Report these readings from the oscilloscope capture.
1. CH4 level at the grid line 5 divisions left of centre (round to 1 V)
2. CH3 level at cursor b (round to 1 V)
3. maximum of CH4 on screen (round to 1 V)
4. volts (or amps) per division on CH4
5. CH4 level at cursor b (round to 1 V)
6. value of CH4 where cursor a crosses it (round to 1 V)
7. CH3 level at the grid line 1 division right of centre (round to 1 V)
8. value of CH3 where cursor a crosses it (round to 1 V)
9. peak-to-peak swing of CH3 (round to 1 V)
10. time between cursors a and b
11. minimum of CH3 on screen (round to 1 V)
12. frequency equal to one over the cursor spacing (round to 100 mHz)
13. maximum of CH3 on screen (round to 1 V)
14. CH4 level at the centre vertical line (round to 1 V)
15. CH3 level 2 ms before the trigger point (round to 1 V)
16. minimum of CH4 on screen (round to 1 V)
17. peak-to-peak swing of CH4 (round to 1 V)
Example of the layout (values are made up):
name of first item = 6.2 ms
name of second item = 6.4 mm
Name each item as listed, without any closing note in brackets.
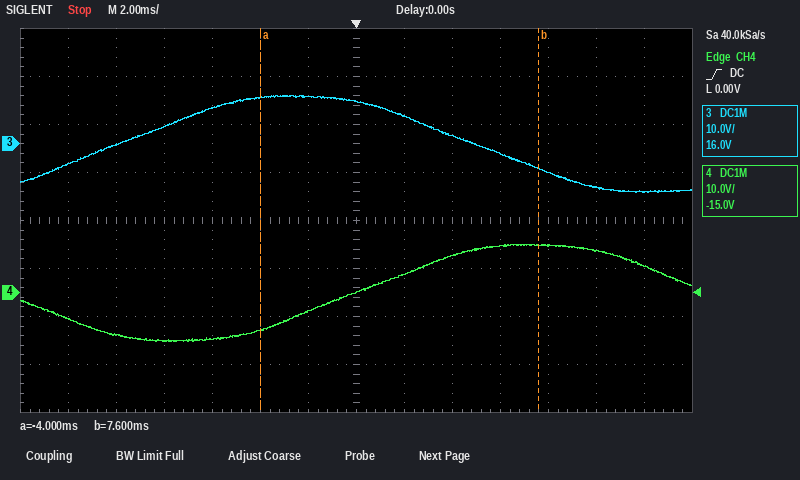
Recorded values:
CH4 level at the grid line 5 divisions left of centre = -9 V
CH3 level at cursor b = -5 V
maximum of CH4 on screen = 10 V
volts (or amps) per division on CH4 = 10 V
CH4 level at cursor b = 10 V
value of CH4 where cursor a crosses it = -8 V
CH3 level at the grid line 1 division right of centre = 6 V
value of CH3 where cursor a crosses it = 10 V
peak-to-peak swing of CH3 = 20 V
time between cursors a and b = 11.6 ms
minimum of CH3 on screen = -10 V
frequency equal to one over the cursor spacing = 86.2 Hz
maximum of CH3 on screen = 10 V
CH4 level at the centre vertical line = 0 V
CH3 level 2 ms before the trigger point = 10 V
minimum of CH4 on screen = -10 V
peak-to-peak swing of CH4 = 20 V
